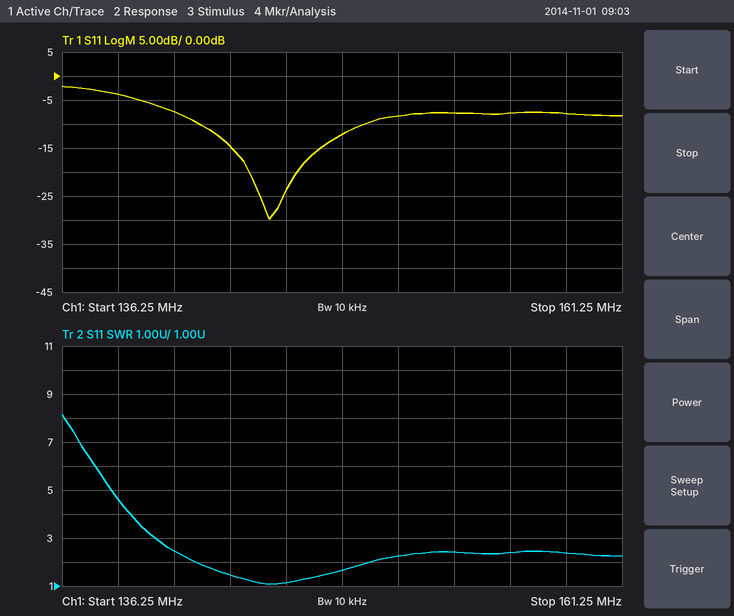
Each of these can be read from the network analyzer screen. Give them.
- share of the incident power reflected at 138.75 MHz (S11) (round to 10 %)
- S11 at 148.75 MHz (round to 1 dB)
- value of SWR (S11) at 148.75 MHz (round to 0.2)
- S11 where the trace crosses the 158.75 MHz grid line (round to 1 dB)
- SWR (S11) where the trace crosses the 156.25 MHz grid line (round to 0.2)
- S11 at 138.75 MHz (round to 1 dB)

40 %
-12 dB
1.6
-8 dB
2.4
-4 dB
